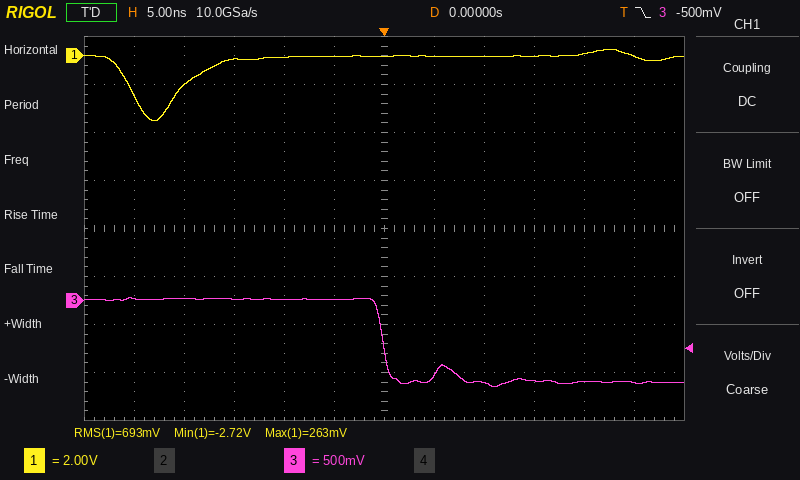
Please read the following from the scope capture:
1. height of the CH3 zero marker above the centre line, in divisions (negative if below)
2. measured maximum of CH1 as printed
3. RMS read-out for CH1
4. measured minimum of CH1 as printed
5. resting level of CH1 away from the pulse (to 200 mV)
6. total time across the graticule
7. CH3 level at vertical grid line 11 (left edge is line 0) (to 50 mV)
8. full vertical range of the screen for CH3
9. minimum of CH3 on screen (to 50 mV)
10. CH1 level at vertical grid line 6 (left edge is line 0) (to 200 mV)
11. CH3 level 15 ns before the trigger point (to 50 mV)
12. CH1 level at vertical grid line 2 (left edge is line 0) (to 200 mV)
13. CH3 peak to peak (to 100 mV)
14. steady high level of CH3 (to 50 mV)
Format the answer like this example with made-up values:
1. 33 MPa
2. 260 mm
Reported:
1. -1.5 div
2. 263 mV
3. 693 mV
4. -2.72 V
5. 0.0 V
6. 60 ns
7. -850 mV
8. 4 V
9. -900 mV
10. 0.0 V
11. 0 mV
12. -1.2 V
13. 900 mV
14. 0 mV
